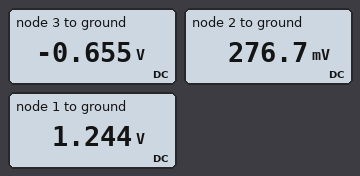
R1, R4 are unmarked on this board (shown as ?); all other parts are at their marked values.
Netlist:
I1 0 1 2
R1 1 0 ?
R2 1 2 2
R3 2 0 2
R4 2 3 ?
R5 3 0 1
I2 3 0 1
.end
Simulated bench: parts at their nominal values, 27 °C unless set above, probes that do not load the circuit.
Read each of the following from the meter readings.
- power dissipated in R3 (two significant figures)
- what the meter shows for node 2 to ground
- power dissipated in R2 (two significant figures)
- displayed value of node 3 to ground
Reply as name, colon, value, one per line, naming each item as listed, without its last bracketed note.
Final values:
power dissipated in R3: 38 mW
what the meter shows for node 2 to ground: 276.7 mV
power dissipated in R2: 470 mW
displayed value of node 3 to ground: -0.655 V
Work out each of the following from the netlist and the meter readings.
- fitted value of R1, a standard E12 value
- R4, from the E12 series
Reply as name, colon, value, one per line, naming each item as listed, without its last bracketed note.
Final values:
fitted value of R1, a standard E12 value: 0.82 Ω
R4, from the E12 series: 2.7 Ω
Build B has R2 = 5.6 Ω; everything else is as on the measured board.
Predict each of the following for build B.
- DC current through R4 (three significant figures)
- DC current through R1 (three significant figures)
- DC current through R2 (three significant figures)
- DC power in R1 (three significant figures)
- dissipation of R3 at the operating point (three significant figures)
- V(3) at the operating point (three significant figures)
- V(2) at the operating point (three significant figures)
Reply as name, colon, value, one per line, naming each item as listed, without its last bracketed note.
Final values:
DC current through R4: 266 mA
DC current through R1: 1.74 A
DC current through R2: 258 mA
DC power in R1: 2.49 W
dissipation of R3 at the operating point: 128 µW
V(3) at the operating point: -734 mV
V(2) at the operating point: -16.0 mV
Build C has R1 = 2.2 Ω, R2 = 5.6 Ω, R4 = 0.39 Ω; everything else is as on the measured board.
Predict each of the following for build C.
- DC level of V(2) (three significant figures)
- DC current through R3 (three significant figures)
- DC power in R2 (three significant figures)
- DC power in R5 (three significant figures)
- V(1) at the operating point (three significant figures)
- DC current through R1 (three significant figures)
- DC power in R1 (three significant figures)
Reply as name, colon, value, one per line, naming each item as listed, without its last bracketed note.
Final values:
DC level of V(2): -115 mV
DC current through R3: 57.6 mA
DC power in R2: 1.88 W
DC power in R5: 132 mW
V(1) at the operating point: 3.13 V
DC current through R1: 1.42 A
DC power in R1: 4.44 W
